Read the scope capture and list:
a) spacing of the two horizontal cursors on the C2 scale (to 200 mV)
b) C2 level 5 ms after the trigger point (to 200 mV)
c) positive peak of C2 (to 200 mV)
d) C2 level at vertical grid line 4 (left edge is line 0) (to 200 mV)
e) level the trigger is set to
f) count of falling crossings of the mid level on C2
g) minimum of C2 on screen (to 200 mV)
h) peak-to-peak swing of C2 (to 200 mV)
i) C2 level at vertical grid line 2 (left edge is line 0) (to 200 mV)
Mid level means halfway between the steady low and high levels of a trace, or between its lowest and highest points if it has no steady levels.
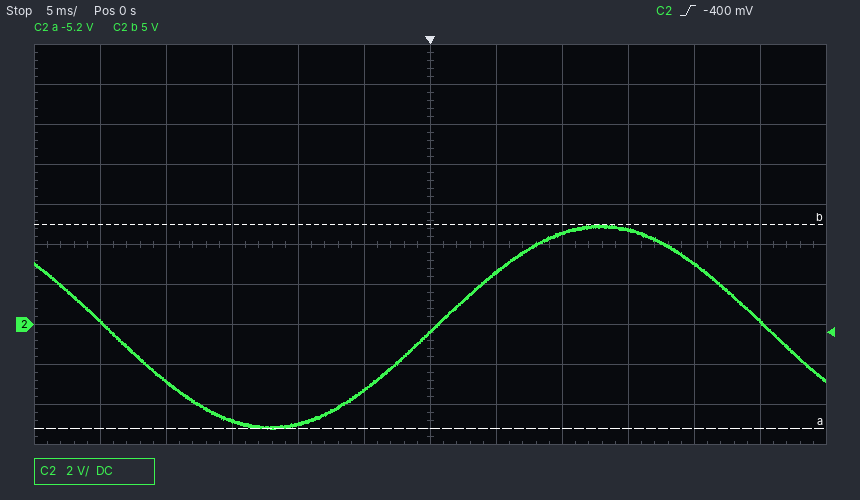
10.2 V
2.6 V
5.0 V
-5.0 V
-400 mV
2
-5.2 V
10.2 V
-2.8 V
